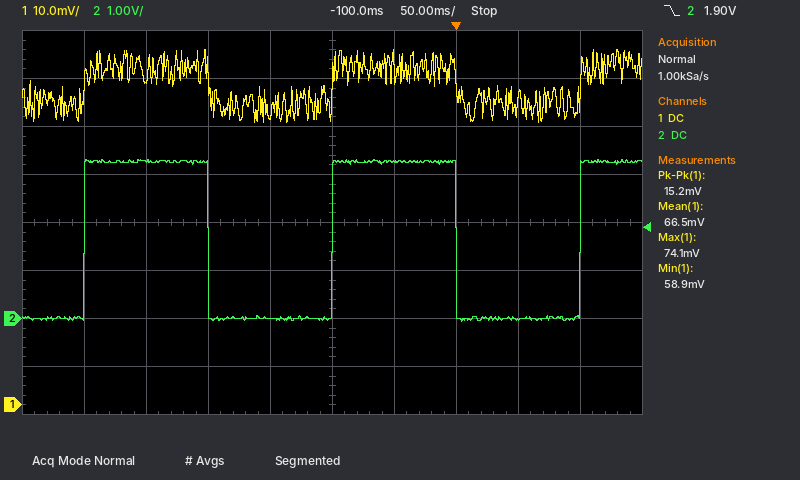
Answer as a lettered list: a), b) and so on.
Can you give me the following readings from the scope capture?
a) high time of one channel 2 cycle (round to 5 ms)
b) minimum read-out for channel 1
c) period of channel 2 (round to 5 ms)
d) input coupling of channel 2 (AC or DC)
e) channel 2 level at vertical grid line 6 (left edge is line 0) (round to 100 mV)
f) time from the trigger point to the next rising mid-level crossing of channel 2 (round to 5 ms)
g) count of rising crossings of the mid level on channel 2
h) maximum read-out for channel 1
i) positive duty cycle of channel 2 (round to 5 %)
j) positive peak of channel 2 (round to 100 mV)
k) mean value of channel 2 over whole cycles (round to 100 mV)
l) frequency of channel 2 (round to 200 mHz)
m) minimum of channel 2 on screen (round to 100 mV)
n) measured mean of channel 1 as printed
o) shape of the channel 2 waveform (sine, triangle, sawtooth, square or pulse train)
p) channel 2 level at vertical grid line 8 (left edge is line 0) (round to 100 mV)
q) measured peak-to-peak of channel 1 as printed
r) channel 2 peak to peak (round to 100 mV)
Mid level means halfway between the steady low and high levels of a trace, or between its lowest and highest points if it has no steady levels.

a) 100 ms
b) 58.9 mV
c) 200 ms
d) DC
e) 3.3 V
f) 100 ms
g) 3
h) 74.1 mV
i) 50 %
j) 3.3 V
k) 1.6 V
l) 5.0 Hz
m) -100 mV
n) 66.5 mV
o) square
p) 0.0 V
q) 15.2 mV
r) 3.4 V
